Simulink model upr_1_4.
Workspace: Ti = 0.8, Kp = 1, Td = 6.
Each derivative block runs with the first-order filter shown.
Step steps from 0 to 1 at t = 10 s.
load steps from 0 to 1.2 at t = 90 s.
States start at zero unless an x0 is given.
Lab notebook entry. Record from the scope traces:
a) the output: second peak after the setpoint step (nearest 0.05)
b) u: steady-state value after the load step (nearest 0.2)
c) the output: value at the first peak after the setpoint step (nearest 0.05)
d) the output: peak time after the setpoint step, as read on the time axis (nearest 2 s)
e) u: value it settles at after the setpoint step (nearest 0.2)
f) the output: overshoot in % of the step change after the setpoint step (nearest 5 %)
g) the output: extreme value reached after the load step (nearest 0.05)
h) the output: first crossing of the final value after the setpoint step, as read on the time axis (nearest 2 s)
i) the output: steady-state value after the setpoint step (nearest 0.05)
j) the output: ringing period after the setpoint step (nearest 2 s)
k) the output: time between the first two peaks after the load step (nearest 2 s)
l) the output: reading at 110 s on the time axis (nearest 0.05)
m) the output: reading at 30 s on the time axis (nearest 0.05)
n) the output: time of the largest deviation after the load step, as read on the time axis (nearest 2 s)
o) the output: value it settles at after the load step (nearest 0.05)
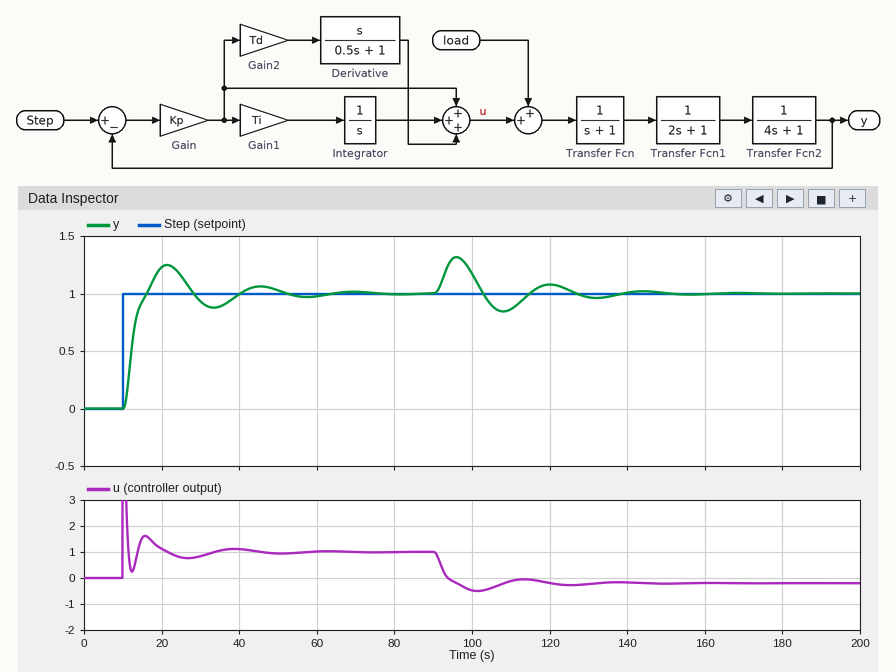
1.05
-0.2
1.25
22 s
1.0
25 %
1.30
16 s
1.00
24 s
24 s
0.85
0.95
96 s
1.00
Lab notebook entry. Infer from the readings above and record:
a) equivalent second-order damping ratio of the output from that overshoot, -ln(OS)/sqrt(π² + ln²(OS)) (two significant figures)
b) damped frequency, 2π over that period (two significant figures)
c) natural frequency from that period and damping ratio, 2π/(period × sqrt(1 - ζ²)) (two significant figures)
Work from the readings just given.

0.40
0.26 rad/s
0.29 rad/s
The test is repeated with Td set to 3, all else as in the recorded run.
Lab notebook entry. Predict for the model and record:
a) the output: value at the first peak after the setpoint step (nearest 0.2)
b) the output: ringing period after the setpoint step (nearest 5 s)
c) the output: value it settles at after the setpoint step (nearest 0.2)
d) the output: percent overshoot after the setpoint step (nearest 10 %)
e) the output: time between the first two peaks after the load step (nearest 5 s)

1.4
20 s
1.0
40 %
20 s
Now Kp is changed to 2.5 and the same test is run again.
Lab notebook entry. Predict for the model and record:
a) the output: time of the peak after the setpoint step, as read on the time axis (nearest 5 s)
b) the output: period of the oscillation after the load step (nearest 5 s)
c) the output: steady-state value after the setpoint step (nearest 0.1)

15 s
20 s
1.0
